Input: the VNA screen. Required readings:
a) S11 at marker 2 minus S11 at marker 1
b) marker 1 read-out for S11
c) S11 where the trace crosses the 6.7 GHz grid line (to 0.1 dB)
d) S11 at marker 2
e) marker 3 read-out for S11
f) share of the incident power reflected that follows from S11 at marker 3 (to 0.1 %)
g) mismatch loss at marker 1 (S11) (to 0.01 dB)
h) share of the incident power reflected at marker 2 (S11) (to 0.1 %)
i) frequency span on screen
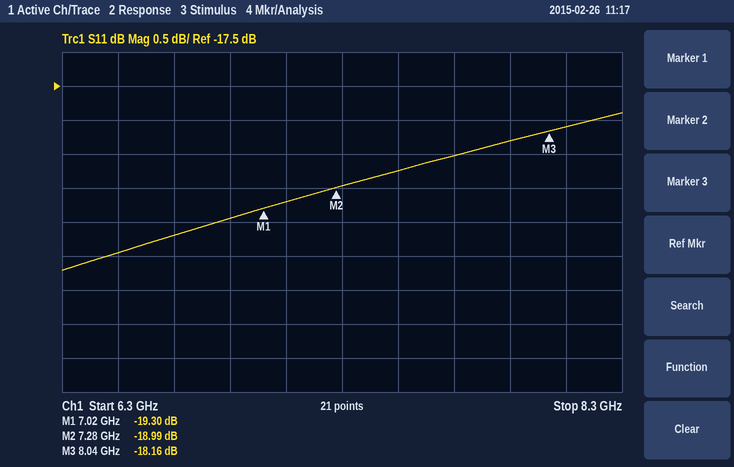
0.31 dB
-19.30 dB
-19.7 dB
-18.99 dB
-18.16 dB
1.5 %
0.05 dB
1.3 %
2 GHz
